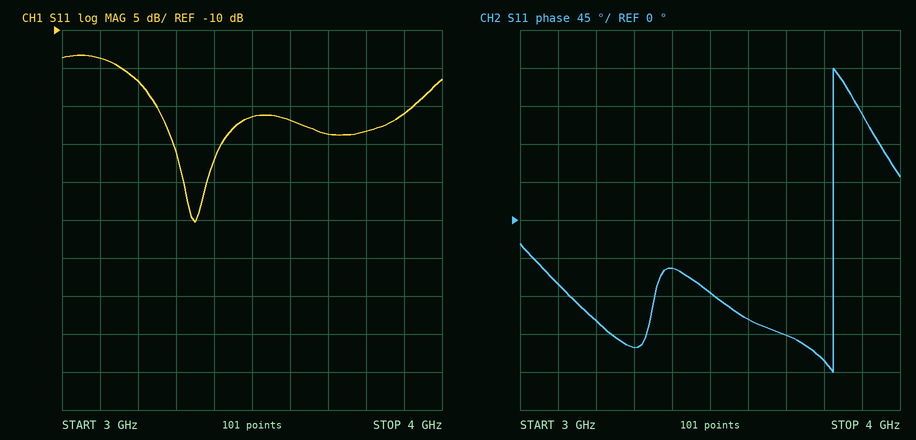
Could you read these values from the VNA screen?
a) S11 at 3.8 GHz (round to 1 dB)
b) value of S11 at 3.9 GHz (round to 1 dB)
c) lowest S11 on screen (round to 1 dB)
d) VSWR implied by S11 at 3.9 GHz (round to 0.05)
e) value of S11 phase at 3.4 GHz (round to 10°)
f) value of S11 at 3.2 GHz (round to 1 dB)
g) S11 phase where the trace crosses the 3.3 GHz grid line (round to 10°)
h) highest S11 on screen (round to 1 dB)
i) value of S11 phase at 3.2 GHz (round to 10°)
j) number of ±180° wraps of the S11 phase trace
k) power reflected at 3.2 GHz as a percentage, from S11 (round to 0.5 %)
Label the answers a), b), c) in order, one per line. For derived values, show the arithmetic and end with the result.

a) -23 dB
b) -21 dB
c) -35 dB
d) |Γ| = 10^(-21/20) = 0.0891; VSWR = (1 + 0.0891)/(1 − 0.0891) ≈ 1.20
e) -60°
f) -17 dB
g) -150°
h) -13 dB
i) -120°
j) 1
k) 10^(-17/10) ≈ 2.0 %
